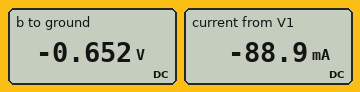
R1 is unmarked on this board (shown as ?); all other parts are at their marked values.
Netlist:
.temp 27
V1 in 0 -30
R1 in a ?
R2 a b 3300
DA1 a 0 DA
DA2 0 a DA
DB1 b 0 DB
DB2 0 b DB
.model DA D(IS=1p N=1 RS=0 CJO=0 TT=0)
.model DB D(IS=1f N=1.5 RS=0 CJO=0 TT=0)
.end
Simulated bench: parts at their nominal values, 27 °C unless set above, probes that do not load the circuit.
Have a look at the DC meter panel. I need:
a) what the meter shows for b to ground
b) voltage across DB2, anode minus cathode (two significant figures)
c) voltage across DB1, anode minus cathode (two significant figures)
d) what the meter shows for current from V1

-0.652 V
650 mV
-650 mV
-88.9 mA
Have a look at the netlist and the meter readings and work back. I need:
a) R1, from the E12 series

330 Ω
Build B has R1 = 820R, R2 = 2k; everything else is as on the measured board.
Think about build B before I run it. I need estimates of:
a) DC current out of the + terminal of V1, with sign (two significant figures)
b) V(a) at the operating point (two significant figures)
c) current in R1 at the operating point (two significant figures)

-36 mA
-630 mV
36 mA
